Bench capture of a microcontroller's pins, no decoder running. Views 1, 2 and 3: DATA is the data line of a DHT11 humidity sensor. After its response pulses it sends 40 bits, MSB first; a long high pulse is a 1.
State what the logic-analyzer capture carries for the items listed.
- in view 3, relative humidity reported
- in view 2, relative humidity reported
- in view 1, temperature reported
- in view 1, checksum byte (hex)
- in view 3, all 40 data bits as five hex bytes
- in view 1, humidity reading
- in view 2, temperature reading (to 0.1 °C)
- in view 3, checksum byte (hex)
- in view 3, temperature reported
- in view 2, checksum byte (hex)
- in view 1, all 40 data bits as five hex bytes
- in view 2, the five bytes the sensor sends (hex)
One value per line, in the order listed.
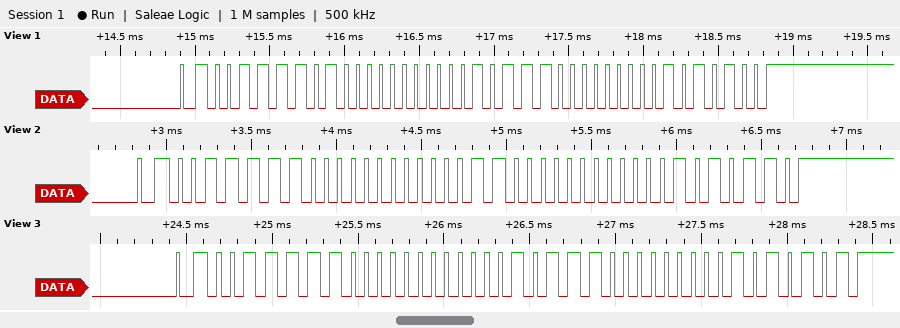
62 %
62 %
23.0 °C
0x54
3E 00 17 00 55
61 %
24.0 °C
0x55
23.0 °C
0x56
3D 00 17 00 54
3E 00 18 00 56
